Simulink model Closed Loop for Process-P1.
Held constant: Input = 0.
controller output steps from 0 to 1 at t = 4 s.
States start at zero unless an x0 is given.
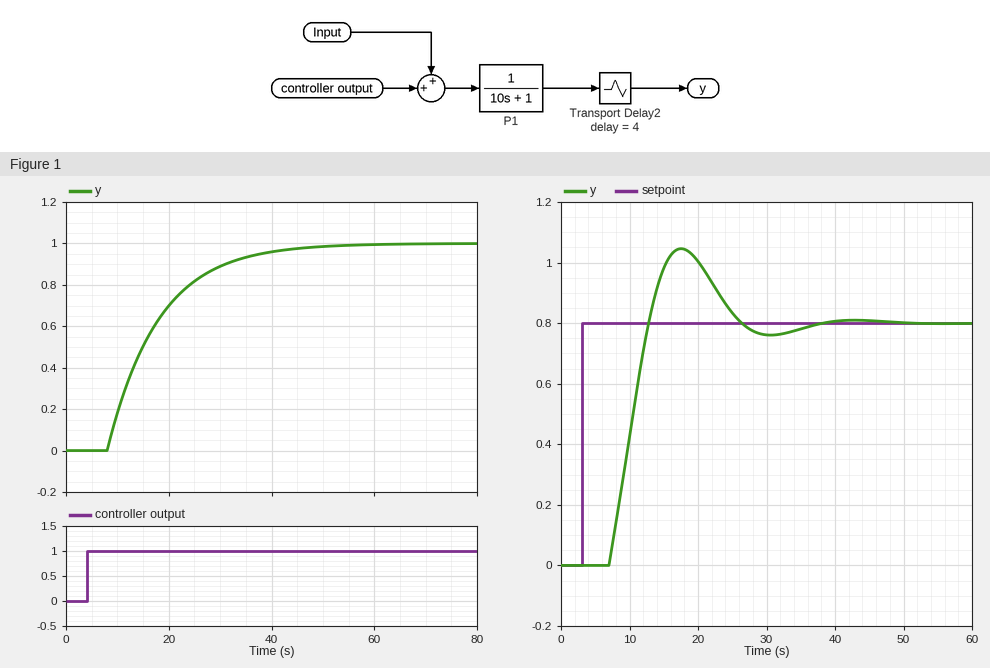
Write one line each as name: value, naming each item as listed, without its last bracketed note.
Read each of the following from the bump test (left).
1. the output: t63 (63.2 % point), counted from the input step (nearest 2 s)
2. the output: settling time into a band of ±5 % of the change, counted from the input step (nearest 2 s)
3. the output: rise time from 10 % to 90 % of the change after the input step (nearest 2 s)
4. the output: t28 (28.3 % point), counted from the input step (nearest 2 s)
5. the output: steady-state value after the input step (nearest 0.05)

the output: t63 (63.2 % point), counted from the input step: 14 s
the output: settling time into a band of ±5 % of the change, counted from the input step: 34 s
the output: rise time from 10 % to 90 % of the change after the input step: 22 s
the output: t28 (28.3 % point), counted from the input step: 8 s
the output: steady-state value after the input step: 1.00
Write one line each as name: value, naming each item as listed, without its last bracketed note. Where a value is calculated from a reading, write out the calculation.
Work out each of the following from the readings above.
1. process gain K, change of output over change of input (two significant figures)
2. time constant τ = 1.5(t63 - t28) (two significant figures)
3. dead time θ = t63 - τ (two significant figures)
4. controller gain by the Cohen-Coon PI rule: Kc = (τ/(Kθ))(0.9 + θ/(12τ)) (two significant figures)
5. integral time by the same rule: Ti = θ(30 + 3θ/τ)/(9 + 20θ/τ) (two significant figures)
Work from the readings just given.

process gain K, change of output over change of input: (1 - 0) / 1 = 1.0
time constant τ = 1.5(t63 - t28): 1.5 × (14 - 8) = 9.0 s
dead time θ = t63 - τ: 14 - 9 = 5.0 s
controller gain by the Cohen-Coon PI rule: Kc = (τ/(Kθ))(0.9 + θ/(12τ)): 9 / (1 × 5) × (0.9 + 5 / (12 × 9)) = 1.7
integral time by the same rule: Ti = θ(30 + 3θ/τ)/(9 + 20θ/τ): 5 × (30 + 3 × 5 / 9) / (9 + 20 × 5 / 9) = 7.9 s
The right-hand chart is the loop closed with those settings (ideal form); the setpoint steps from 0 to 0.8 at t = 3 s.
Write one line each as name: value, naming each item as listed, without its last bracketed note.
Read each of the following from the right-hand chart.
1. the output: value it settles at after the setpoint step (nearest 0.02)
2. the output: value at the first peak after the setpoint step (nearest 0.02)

the output: value it settles at after the setpoint step: 0.80
the output: value at the first peak after the setpoint step: 1.04
